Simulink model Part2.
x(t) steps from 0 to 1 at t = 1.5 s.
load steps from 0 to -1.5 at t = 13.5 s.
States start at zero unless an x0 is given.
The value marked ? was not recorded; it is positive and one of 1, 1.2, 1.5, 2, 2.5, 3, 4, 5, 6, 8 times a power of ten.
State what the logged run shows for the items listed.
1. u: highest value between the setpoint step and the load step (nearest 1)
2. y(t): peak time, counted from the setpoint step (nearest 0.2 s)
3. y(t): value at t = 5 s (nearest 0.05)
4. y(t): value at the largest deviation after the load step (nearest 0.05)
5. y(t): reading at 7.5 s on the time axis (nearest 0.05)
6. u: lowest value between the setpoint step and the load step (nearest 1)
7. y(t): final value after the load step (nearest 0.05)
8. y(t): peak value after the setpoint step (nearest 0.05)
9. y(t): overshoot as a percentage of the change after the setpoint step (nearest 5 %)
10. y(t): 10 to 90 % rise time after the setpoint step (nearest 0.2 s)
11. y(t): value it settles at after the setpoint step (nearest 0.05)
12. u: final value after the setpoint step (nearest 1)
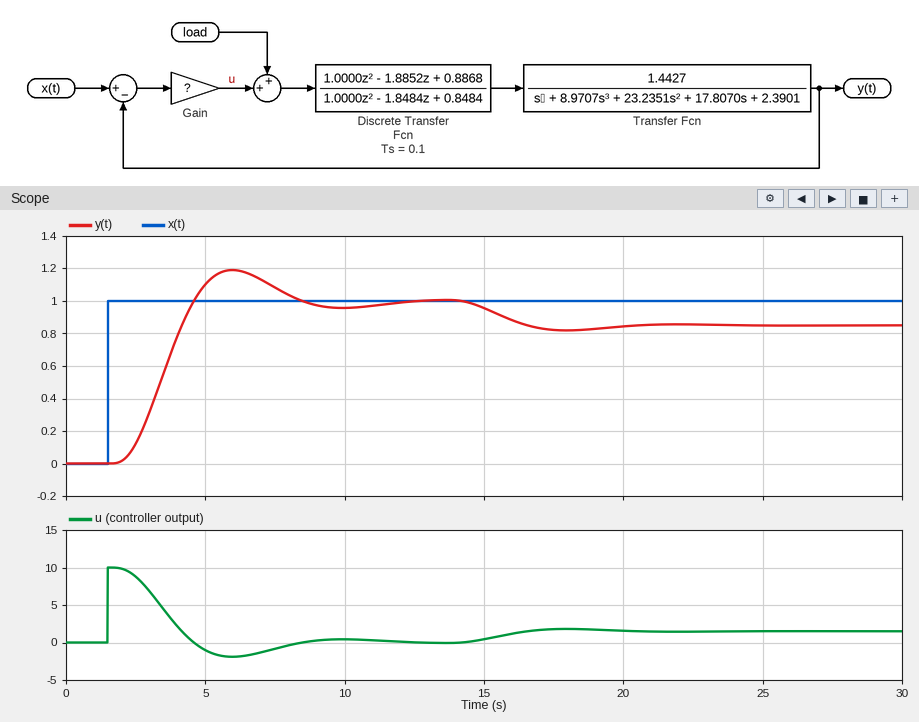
10
4.4 s
1.10
0.80
1.10
-2
0.85
1.20
20 %
1.8 s
1.00
0
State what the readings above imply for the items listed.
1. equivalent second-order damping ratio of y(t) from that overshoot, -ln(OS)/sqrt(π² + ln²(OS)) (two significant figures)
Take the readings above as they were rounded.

0.46
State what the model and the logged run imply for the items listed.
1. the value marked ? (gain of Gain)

10
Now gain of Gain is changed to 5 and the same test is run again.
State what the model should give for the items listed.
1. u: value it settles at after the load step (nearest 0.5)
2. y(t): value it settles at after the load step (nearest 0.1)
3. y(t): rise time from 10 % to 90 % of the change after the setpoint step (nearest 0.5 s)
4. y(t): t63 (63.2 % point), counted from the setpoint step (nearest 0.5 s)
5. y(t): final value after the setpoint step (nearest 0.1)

1.5
0.7
4.0 s
3.5 s
1.0
